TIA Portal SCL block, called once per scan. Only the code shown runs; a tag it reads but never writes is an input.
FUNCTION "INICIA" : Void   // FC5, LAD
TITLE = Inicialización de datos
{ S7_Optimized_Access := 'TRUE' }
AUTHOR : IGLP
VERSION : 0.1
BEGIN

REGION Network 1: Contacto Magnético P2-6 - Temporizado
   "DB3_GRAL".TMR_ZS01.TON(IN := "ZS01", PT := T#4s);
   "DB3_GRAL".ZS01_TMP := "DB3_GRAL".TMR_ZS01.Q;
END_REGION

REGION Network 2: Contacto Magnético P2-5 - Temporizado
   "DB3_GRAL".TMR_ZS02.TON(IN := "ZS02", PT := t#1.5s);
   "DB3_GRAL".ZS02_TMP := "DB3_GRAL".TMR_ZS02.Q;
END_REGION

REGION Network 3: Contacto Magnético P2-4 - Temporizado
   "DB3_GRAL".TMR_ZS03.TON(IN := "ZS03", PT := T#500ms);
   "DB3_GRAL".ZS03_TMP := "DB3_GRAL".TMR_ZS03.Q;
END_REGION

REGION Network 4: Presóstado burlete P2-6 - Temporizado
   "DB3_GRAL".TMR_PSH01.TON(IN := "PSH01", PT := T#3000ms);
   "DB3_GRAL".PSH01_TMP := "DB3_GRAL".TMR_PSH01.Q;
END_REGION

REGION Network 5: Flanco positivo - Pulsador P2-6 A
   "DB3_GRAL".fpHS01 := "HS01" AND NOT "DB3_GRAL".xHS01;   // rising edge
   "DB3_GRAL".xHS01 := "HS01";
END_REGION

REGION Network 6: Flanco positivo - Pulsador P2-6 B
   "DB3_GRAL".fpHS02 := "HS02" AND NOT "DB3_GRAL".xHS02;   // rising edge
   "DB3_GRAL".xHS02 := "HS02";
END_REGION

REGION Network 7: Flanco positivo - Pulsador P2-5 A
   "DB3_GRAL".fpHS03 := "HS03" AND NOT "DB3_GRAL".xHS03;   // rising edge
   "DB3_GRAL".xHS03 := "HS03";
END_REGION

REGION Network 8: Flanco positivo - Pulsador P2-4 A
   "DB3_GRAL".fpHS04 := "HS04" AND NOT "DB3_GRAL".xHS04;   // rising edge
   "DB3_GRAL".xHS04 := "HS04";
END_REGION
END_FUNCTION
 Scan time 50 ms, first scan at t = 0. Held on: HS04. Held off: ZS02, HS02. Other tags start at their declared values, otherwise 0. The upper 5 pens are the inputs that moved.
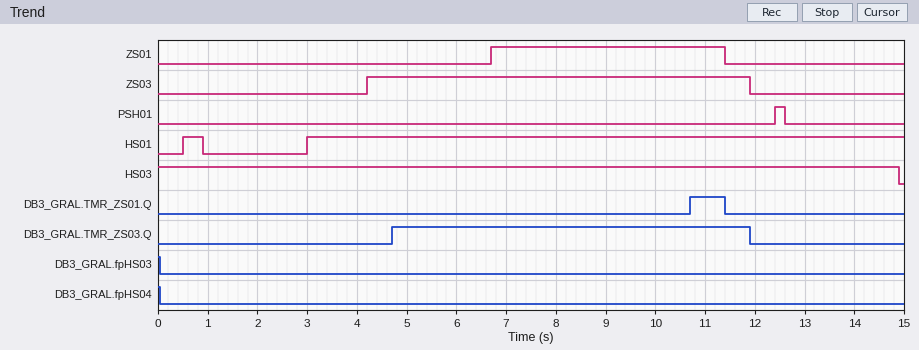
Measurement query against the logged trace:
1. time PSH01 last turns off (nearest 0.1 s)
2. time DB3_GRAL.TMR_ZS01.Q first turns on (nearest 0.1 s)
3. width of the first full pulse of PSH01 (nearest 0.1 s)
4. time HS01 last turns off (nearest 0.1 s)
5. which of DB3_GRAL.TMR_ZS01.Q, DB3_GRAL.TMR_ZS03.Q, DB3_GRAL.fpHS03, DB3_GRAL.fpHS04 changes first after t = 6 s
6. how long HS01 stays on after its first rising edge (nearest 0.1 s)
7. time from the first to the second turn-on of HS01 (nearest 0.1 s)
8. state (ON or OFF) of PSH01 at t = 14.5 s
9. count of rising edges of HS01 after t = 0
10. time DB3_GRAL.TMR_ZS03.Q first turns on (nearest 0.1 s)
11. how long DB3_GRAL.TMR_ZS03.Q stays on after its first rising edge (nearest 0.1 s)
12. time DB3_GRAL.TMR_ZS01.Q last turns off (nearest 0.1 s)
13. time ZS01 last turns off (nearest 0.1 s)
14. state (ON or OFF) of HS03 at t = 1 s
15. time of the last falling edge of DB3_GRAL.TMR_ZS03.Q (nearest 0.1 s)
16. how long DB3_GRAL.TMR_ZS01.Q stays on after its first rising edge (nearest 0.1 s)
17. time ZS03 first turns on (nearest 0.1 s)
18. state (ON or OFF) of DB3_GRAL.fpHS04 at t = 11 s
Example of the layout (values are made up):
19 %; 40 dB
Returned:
12.6 s; 10.7 s; 0.2 s; 0.9 s; DB3_GRAL.TMR_ZS01.Q; 0.4 s; 2.5 s; OFF; 2; 4.7 s; 7.2 s; 11.4 s; 11.4 s; ON; 11.9 s; 0.7 s; 4.2 s; OFF
